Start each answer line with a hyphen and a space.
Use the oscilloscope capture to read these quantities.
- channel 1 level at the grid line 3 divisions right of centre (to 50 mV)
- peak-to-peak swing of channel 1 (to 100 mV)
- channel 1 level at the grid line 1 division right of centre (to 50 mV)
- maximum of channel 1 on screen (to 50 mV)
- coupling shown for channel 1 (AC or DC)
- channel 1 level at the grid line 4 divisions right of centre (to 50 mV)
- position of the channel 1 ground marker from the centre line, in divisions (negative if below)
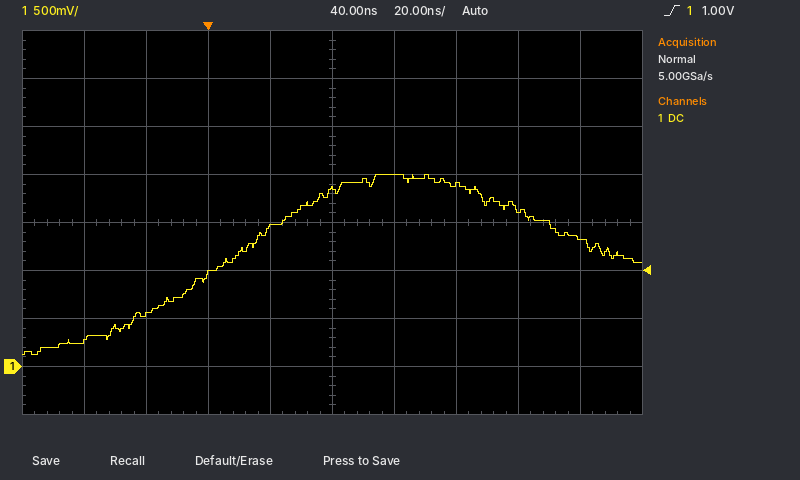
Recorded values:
- 1.65 V
- 1.90 V
- 2.00 V
- 2.00 V
- DC
- 1.35 V
- -3.0 div
